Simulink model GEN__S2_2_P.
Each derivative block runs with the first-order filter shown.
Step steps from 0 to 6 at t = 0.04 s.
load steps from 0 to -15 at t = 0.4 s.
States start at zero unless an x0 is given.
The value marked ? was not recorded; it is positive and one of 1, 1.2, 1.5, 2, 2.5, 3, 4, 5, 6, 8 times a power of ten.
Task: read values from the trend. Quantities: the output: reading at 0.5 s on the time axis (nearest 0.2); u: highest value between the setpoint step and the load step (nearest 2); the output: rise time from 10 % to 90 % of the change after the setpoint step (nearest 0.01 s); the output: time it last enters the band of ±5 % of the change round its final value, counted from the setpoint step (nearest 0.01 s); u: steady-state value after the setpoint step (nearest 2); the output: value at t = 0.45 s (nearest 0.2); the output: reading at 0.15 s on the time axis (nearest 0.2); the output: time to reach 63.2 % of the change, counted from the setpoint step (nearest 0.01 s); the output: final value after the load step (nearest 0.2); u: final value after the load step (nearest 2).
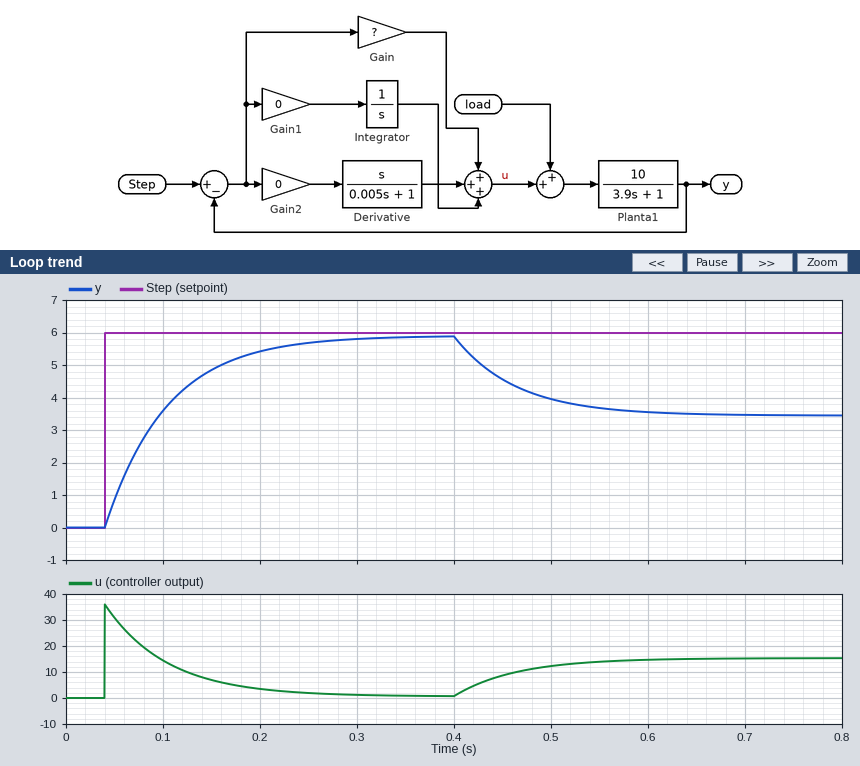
4.0
36
0.14 s
0.19 s
0
4.6
4.8
0.06 s
3.4
16
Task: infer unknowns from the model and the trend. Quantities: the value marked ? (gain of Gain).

6
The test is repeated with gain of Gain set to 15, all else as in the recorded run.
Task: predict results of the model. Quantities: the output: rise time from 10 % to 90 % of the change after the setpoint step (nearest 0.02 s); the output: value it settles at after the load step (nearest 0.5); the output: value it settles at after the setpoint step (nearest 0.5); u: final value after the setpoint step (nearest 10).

0.06 s
5.0
6.0
0
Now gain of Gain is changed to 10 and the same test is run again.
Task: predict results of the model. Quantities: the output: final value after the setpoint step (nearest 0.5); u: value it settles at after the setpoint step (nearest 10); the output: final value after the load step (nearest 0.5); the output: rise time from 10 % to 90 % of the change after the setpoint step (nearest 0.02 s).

6.0
0
4.5
0.08 s
